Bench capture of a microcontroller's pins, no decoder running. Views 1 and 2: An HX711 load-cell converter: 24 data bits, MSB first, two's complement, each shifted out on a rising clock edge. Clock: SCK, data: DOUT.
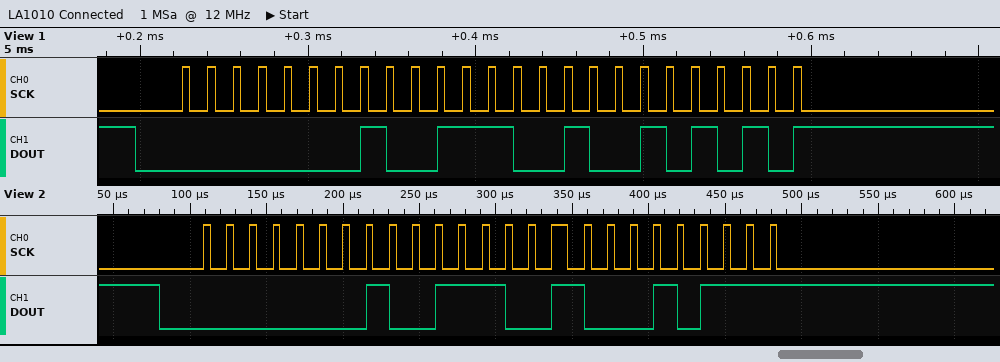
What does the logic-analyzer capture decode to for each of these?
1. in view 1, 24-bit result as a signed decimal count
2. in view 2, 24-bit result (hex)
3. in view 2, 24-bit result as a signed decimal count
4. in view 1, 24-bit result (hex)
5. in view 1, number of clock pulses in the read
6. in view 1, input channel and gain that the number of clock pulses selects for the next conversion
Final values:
80170
0x013917
80151
0x01392A
25
channel A, gain 128
